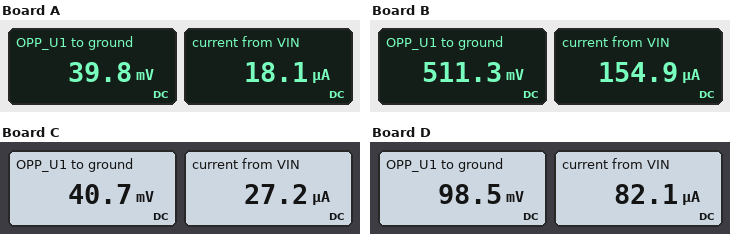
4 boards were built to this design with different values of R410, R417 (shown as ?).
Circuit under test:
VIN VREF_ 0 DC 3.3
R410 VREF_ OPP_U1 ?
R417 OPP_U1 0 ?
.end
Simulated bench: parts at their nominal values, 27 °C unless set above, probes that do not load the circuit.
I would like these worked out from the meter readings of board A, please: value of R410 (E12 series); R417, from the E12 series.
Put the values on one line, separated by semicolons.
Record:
180 kΩ; 2.2 kΩ
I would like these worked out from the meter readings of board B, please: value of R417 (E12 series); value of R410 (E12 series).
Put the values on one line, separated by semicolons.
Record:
3.3 kΩ; 18 kΩ
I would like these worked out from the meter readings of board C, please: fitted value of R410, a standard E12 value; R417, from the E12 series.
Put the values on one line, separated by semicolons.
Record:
120 kΩ; 1.5 kΩ
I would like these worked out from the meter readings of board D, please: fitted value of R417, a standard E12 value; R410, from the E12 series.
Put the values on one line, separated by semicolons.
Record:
1.2 kΩ; 39 kΩ
